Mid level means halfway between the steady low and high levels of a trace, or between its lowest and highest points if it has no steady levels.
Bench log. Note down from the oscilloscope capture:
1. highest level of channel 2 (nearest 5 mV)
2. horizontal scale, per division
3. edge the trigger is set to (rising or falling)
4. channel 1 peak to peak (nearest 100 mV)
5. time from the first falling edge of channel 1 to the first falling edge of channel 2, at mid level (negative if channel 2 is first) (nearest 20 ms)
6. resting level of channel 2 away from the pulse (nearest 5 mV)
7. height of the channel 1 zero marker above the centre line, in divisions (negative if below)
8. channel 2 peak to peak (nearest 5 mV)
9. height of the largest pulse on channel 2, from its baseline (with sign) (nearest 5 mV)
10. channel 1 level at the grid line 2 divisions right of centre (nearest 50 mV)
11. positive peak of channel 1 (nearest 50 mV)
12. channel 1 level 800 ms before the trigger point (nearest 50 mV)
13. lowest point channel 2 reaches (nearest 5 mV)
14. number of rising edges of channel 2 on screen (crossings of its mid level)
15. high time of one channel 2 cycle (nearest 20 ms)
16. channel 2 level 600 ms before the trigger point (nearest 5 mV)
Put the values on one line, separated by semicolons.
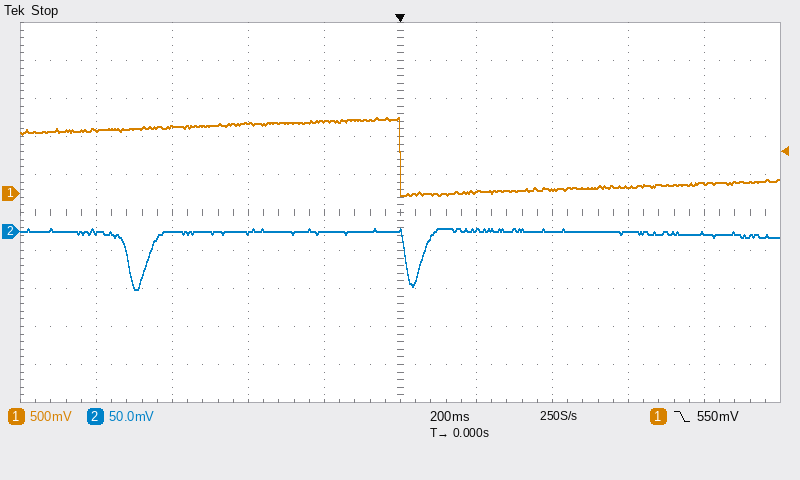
5 mV; 200 ms; falling; 1.00 V; -720 ms; 0 mV; +0.5 div; 80 mV; -75 mV; 50 mV; 1.00 V; 850 mV; -75 mV; 2; 680 ms; 0 mV
